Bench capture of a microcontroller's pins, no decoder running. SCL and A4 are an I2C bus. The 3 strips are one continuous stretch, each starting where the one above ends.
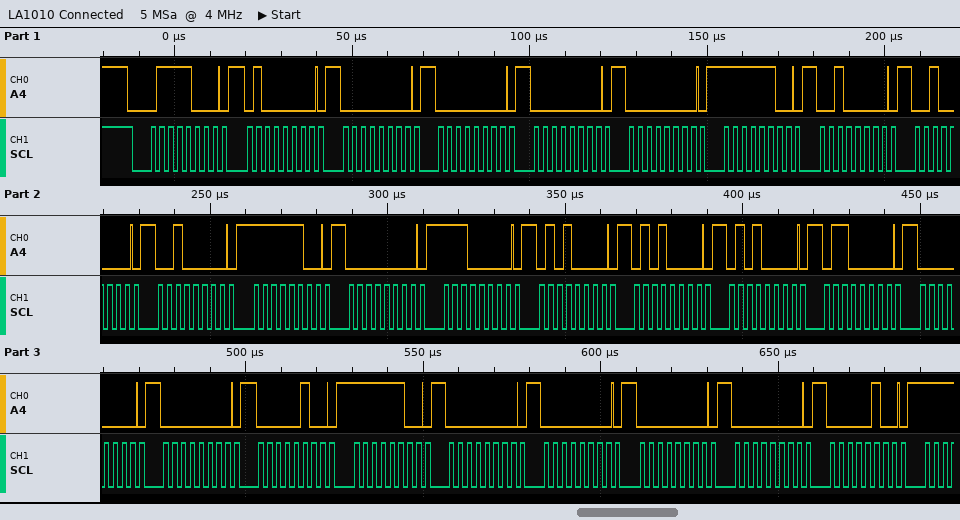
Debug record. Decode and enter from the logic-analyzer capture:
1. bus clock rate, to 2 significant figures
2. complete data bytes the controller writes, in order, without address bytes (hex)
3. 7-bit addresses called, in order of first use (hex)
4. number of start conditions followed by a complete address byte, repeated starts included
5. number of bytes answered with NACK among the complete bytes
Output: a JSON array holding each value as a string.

["400 kHz", "40 00 00 00 00 FC 20 20 20 FC 00 E0 50 50 50 60 00 00 04 FC 00 00 00 00 04", "0x3C", "1", "0"]
